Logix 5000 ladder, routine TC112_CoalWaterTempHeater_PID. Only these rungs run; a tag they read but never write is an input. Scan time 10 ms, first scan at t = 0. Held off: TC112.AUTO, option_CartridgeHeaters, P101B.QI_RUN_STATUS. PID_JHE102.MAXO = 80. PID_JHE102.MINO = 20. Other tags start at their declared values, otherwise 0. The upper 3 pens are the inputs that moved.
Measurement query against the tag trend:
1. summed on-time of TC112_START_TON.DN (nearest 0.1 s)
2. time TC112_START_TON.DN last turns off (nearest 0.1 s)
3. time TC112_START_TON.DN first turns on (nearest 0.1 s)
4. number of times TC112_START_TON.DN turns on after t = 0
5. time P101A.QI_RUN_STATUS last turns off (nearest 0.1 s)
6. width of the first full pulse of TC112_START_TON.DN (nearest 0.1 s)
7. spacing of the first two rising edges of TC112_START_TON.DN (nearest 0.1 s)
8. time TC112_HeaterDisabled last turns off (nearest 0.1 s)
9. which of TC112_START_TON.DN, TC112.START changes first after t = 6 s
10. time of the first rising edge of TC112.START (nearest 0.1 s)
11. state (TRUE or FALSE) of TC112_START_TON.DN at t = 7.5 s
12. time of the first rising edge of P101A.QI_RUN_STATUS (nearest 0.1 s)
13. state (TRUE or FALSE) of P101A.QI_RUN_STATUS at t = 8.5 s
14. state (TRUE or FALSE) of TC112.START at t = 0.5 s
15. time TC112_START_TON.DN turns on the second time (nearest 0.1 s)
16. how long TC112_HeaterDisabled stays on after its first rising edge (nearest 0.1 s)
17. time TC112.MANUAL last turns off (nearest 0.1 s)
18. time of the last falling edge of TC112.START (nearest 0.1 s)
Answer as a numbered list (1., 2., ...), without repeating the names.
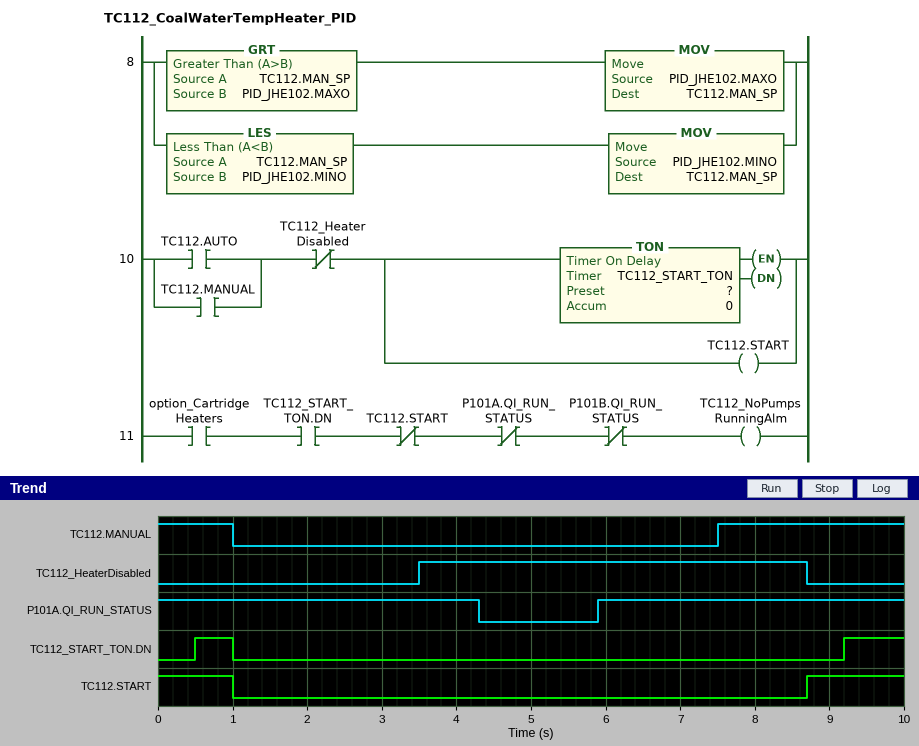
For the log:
1. 1.3 s
2. 1.0 s
3. 0.5 s
4. 2
5. 4.3 s
6. 0.5 s
7. 8.7 s
8. 8.7 s
9. TC112.START
10. 8.7 s
11. FALSE
12. 5.9 s
13. TRUE
14. TRUE
15. 9.2 s
16. 5.2 s
17. 1.0 s
18. 1.0 s
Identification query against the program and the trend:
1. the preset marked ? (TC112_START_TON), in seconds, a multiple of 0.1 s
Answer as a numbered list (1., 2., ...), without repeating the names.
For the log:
1. 0.5 s
